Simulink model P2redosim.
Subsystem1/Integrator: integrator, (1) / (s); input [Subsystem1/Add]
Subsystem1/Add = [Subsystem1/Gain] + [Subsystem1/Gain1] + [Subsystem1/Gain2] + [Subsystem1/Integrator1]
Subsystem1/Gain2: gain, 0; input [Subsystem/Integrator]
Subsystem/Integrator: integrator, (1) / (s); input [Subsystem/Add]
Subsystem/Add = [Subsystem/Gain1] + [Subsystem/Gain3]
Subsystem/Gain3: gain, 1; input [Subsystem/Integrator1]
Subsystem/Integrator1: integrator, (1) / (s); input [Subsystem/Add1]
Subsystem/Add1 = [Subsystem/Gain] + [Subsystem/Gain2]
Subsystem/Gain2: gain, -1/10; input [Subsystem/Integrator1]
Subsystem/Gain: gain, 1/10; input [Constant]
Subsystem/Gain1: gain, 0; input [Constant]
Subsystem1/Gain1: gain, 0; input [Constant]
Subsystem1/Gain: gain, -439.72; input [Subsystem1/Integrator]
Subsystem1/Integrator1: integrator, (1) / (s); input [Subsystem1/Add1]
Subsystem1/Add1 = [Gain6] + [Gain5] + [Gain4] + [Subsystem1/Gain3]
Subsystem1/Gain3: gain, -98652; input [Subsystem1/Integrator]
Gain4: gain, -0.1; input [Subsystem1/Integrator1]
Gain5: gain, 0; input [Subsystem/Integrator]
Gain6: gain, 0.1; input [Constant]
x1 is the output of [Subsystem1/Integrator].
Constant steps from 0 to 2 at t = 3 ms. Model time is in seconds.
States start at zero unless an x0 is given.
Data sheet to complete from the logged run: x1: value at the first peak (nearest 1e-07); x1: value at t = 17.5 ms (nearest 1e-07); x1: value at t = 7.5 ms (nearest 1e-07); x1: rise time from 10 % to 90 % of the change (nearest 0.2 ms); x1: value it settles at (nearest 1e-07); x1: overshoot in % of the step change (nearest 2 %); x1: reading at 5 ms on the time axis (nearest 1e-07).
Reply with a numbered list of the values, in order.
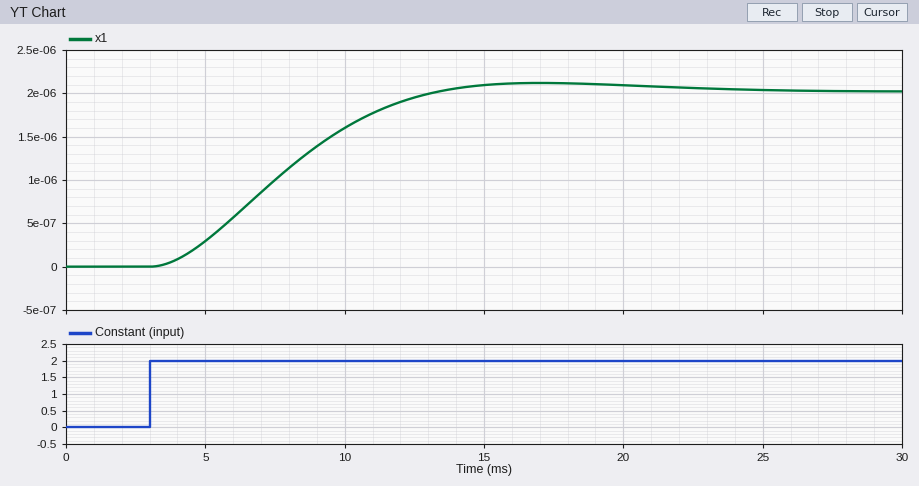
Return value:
1. 0.0000021
2. 0.0000021
3. 0.0000010
4. 6.8 ms
5. 0.0000020
6. 4 %
7. 0.0000003
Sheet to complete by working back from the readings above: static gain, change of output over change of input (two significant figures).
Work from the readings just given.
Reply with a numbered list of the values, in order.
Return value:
1. 0.0000010
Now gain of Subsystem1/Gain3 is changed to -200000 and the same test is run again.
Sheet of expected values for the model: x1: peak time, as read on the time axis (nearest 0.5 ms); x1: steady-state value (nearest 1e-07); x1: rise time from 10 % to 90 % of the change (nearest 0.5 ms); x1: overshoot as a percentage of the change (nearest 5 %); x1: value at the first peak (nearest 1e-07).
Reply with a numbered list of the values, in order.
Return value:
1. 11.0 ms
2. 0.0000010
3. 3.5 ms
4. 15 %
5. 0.0000012
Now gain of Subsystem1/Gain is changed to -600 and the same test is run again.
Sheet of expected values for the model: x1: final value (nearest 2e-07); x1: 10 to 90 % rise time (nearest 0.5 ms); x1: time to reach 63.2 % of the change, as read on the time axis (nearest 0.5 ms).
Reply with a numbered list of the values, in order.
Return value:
1. 0.0000020
2. 10.0 ms
3. 9.5 ms
